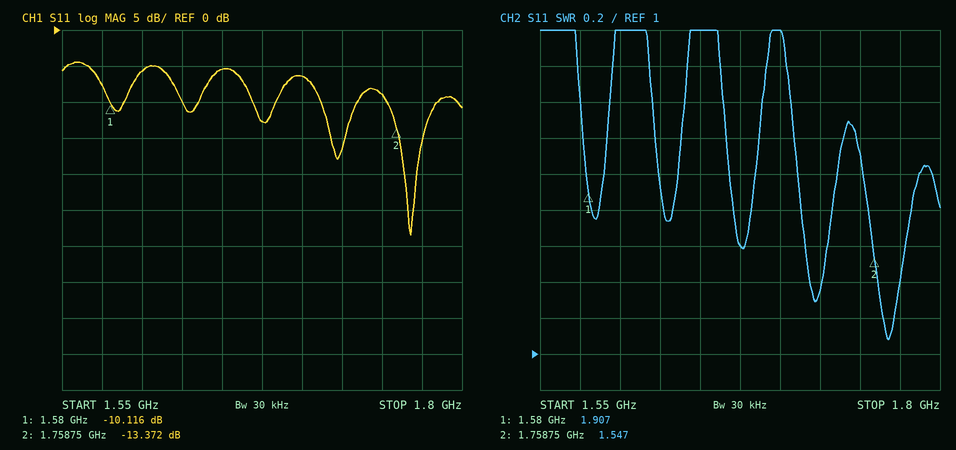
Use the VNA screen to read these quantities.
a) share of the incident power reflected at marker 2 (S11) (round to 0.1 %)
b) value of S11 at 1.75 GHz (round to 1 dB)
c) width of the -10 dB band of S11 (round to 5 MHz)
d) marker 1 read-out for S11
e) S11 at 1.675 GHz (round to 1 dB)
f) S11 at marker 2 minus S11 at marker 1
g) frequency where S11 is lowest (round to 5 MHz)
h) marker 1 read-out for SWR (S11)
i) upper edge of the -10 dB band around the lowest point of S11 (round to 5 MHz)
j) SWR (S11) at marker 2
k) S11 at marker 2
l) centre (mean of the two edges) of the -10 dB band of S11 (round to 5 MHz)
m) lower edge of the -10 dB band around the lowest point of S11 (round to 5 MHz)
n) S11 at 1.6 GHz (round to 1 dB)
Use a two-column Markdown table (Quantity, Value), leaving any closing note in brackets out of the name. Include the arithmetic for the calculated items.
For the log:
| Quantity | Value |
|---|---|
| share of the incident power reflected at marker 2 (S11) | 10^(-13.372/10) ≈ 4.6 % |
| value of S11 at 1.75 GHz | -9 dB |
| width of the -10 dB band of S11 | 1.785 GHz − 1.755 GHz = 30 MHz |
| marker 1 read-out for S11 | -10.116 dB |
| S11 at 1.675 GHz | -13 dB |
| S11 at marker 2 minus S11 at marker 1 | -13.372 − (-10.116) = -3.256 dB |
| frequency where S11 is lowest | 1.770 GHz |
| marker 1 read-out for SWR | 1.907 |
| upper edge of the -10 dB band around the lowest point of S11 | 1.785 GHz |
| SWR (S11) at marker 2 | 1.547 |
| S11 at marker 2 | -13.372 dB |
| centre (mean of the two edges) of the -10 dB band of S11 | 1.770 GHz |
| lower edge of the -10 dB band around the lowest point of S11 | 1.755 GHz |
| S11 at 1.6 GHz | -6 dB |
